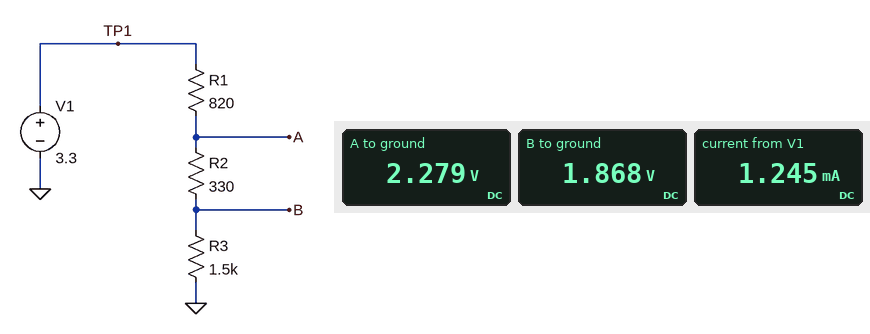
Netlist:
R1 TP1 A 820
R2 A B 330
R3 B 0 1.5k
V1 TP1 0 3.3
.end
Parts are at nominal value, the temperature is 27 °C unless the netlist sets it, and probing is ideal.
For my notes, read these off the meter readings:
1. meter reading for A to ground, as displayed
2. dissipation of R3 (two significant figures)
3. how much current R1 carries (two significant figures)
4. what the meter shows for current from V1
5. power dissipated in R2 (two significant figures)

2.279 V
2.3 mW
1.2 mA
1.245 mA
510 µW
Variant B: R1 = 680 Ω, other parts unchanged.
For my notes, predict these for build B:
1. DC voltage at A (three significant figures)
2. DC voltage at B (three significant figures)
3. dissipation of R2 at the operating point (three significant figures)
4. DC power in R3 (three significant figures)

2.41 V
1.97 V
570 µW
2.59 mW
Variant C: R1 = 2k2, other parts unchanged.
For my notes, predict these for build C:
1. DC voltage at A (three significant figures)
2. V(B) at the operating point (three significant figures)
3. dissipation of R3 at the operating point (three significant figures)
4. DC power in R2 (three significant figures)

1.50 V
1.23 V
1.01 mW
221 µW
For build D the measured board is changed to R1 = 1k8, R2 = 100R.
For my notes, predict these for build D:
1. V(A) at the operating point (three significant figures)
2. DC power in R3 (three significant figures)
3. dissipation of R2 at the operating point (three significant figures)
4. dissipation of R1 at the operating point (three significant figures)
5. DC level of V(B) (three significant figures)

1.55 V
1.41 mW
94.2 µW
1.70 mW
1.46 V
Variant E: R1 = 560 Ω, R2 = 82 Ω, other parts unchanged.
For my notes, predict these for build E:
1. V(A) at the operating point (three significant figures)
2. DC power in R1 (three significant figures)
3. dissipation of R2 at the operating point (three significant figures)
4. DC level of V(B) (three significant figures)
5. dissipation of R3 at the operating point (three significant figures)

2.44 V
1.33 mW
195 µW
2.31 V
3.56 mW
